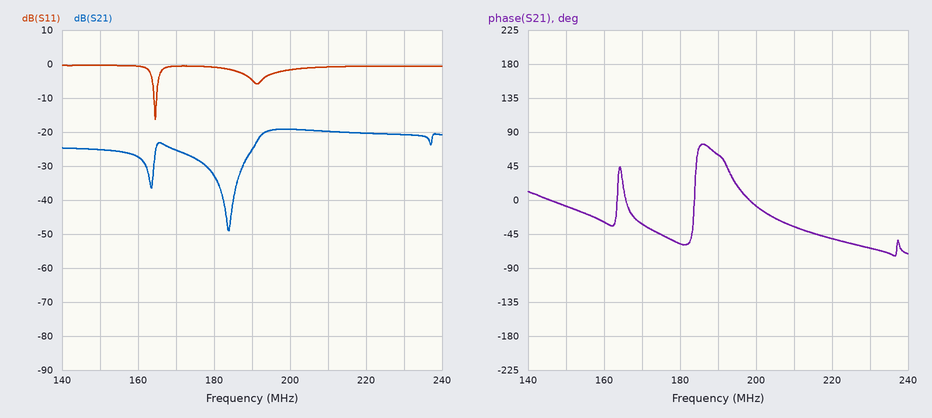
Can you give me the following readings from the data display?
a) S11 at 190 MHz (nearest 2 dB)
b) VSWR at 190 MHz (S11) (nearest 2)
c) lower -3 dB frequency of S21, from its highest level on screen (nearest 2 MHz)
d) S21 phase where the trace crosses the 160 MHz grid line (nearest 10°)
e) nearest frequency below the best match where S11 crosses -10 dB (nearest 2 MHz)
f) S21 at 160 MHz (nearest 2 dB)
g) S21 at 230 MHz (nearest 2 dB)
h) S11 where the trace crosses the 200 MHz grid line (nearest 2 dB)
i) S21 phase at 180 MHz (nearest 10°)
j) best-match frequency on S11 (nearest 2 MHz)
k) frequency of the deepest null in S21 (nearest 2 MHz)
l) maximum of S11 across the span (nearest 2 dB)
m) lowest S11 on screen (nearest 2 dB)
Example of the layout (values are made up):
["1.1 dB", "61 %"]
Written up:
["-4 dB", "4", "192 MHz", "-30°", "164 MHz", "-28 dB", "-20 dB", "-2 dB", "-60°", "164 MHz", "184 MHz", "0 dB", "-16 dB"]
